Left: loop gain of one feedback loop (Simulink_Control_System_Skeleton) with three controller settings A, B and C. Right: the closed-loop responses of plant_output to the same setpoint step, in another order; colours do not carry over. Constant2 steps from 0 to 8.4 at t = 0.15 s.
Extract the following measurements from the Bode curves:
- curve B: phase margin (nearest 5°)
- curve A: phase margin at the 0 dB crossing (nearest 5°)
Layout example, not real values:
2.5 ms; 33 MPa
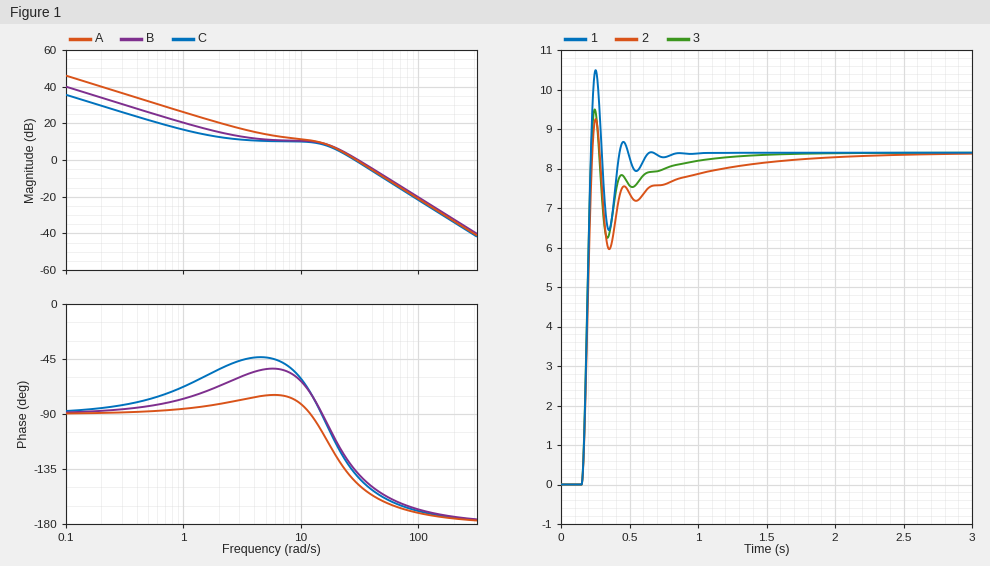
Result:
40°; 35°
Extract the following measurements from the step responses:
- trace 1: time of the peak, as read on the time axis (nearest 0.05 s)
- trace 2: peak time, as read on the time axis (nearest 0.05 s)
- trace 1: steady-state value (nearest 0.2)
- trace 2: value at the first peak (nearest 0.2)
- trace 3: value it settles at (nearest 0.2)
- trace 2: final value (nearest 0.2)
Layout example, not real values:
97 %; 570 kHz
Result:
0.25 s; 0.25 s; 8.4; 9.2; 8.4; 8.4
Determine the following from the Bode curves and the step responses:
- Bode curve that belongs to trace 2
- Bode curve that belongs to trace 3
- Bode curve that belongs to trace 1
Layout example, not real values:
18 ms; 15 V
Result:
C; B; A
